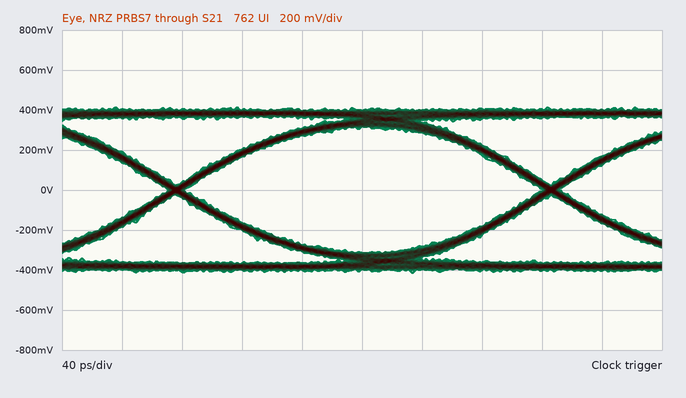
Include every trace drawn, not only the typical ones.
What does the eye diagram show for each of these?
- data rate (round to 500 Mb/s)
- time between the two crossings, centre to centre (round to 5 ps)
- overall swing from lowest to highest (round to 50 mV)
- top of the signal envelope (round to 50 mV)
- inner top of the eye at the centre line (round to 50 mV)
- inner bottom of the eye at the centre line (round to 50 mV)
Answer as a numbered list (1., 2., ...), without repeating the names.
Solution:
1. 4.0 Gb/s
2. 250 ps
3. 850 mV
4. 400 mV
5. 300 mV
6. -300 mV
